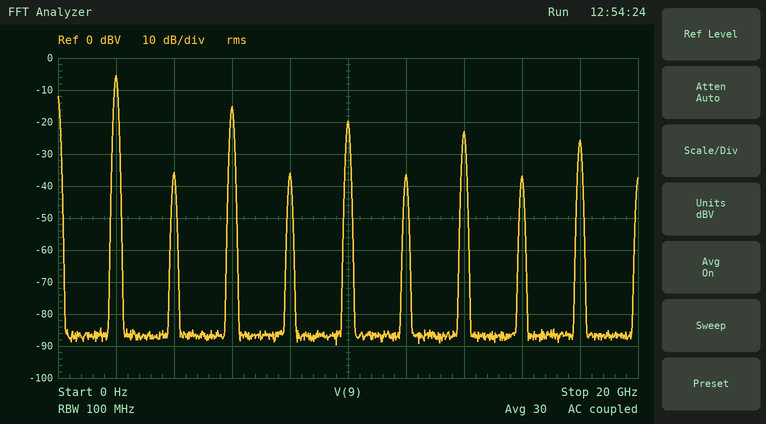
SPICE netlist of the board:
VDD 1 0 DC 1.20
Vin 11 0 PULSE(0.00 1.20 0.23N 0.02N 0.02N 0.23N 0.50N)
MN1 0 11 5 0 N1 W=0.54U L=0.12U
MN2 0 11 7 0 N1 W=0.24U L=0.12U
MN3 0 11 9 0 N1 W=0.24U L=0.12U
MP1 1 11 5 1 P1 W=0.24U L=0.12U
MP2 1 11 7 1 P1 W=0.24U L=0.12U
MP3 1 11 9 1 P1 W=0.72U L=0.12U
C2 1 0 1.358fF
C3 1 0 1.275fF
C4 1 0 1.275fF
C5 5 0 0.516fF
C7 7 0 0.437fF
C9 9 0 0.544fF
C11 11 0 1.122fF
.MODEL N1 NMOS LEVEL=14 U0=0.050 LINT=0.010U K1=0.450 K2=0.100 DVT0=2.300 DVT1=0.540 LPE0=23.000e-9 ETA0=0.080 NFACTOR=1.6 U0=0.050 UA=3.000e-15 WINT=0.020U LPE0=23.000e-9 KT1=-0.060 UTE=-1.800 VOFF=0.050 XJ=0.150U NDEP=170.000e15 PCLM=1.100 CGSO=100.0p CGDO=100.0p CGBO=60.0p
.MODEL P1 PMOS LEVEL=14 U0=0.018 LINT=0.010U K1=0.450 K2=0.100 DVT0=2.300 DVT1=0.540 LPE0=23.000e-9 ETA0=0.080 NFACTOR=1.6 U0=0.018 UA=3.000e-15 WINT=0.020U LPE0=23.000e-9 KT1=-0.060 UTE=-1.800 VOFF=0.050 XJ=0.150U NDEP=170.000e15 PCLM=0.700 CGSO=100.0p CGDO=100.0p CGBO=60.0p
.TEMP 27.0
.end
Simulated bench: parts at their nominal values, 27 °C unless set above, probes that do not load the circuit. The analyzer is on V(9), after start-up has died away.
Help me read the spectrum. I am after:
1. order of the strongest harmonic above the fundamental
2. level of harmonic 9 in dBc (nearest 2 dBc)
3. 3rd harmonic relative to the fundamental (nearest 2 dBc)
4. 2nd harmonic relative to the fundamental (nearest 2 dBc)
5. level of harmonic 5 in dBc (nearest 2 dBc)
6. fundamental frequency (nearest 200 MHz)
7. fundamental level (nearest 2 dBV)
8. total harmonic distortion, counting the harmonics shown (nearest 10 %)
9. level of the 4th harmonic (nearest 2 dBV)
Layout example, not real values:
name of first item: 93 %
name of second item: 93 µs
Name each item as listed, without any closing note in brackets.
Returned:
order of the strongest harmonic above the fundamental: 3
level of harmonic 9 in dBc: -20 dBc
3rd harmonic relative to the fundamental: -10 dBc
2nd harmonic relative to the fundamental: -30 dBc
level of harmonic 5 in dBc: -14 dBc
fundamental frequency: 2.0 GHz
fundamental level: -6 dBV
total harmonic distortion, counting the harmonics shown: 40 %
level of the 4th harmonic: -36 dBV
